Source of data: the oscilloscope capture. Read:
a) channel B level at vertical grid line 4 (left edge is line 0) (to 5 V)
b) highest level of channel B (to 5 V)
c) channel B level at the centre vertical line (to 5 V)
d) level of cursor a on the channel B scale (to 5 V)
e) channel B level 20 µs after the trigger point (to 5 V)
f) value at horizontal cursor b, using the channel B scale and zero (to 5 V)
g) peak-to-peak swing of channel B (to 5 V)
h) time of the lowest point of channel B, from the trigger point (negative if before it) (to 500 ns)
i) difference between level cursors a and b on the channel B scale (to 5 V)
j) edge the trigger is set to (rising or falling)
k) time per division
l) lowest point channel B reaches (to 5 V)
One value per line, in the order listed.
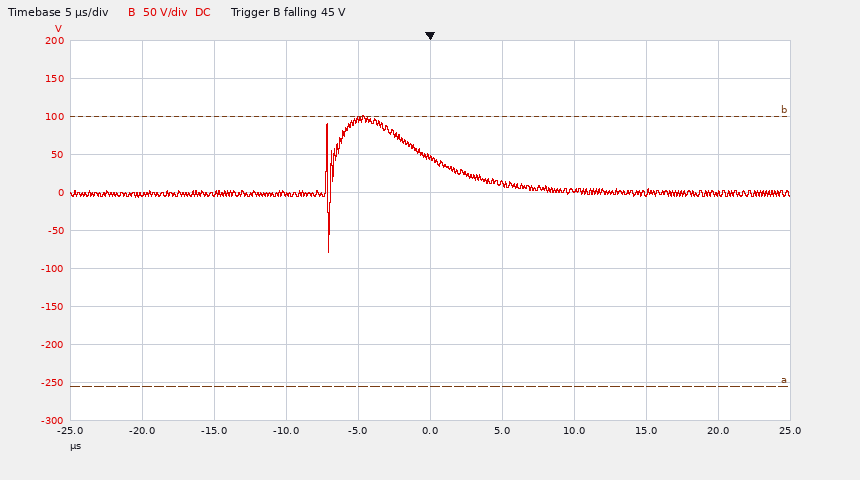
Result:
95 V
100 V
45 V
-255 V
0 V
100 V
180 V
-7.0 µs
355 V
falling
5 µs
-80 V
